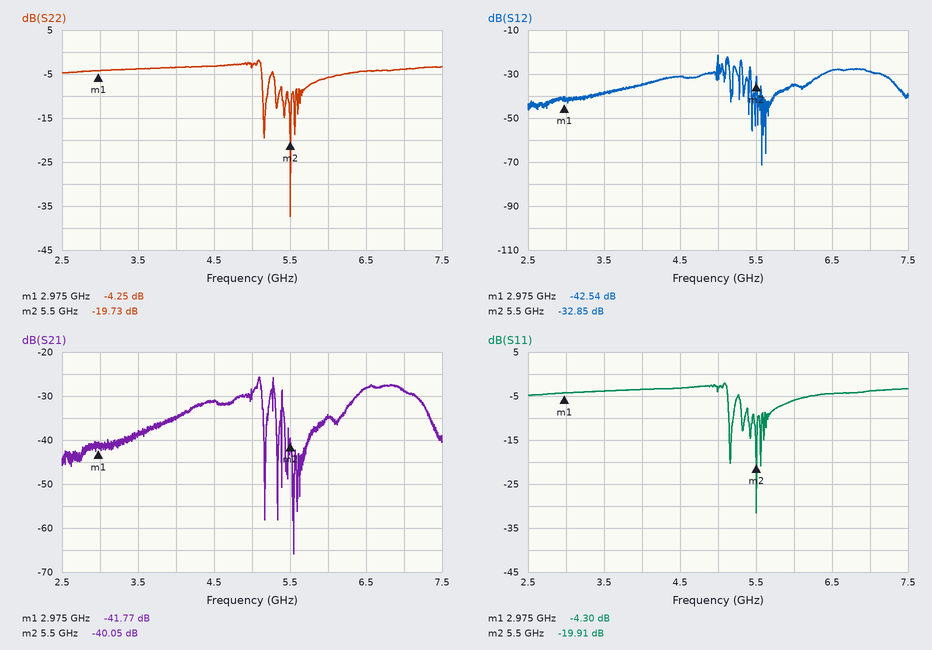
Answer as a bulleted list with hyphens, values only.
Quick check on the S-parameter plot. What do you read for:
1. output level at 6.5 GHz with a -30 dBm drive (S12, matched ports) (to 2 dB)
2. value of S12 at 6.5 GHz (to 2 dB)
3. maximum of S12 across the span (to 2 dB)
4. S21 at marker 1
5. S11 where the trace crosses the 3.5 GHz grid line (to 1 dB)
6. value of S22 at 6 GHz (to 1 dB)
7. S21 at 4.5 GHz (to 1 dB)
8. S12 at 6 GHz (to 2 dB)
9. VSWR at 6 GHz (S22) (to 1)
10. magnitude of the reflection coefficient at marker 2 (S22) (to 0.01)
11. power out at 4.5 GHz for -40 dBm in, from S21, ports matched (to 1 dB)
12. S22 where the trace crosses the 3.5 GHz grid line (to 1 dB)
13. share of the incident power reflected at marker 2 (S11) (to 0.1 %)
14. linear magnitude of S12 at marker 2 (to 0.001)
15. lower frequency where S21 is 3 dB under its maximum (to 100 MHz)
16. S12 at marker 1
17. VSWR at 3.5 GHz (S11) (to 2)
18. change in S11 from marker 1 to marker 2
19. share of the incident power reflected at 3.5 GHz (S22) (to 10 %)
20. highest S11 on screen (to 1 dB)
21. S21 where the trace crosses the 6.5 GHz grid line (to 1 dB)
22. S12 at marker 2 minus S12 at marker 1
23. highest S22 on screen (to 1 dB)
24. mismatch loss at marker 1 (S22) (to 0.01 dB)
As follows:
- -58 dBm
- -28 dB
- -22 dB
- -41.77 dB
- -4 dB
- -6 dB
- -31 dB
- -36 dB
- 3
- 0.10
- -71 dBm
- -4 dB
- 1.0 %
- 0.023
- 5.0 GHz
- -42.54 dB
- 4
- -15.61 dB
- 40 %
- -2 dB
- -28 dB
- 9.69 dB
- -2 dB
- 2.05 dB
